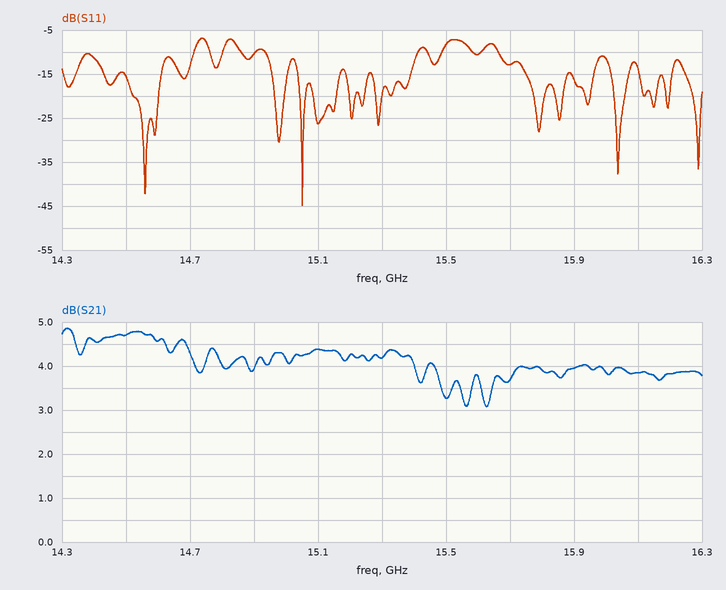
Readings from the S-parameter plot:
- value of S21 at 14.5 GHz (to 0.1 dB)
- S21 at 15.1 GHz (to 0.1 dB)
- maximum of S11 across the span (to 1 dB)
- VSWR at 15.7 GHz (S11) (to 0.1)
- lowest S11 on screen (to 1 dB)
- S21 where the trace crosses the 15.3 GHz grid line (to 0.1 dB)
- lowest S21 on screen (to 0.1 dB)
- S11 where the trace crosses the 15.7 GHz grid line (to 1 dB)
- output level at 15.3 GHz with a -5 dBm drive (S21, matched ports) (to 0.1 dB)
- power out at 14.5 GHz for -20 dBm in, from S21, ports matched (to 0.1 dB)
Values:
4.7 dB
4.4 dB
-7 dB
1.6
-45 dB
4.2 dB
3.1 dB
-13 dB
-0.8 dBm
-15.3 dBm
